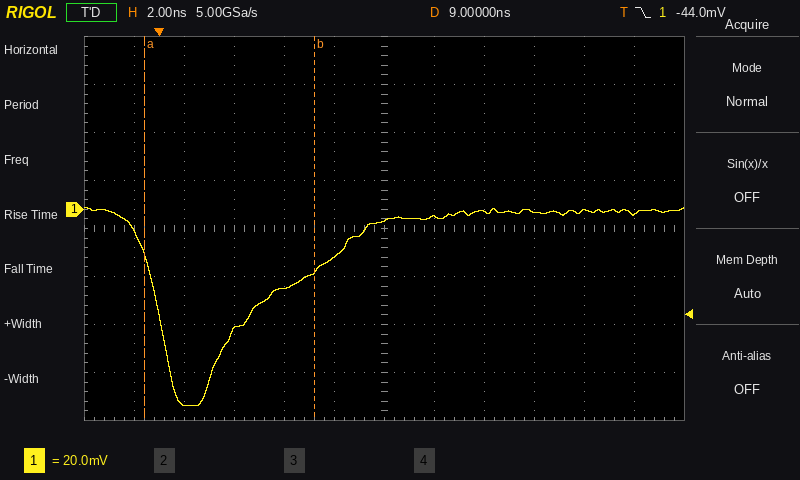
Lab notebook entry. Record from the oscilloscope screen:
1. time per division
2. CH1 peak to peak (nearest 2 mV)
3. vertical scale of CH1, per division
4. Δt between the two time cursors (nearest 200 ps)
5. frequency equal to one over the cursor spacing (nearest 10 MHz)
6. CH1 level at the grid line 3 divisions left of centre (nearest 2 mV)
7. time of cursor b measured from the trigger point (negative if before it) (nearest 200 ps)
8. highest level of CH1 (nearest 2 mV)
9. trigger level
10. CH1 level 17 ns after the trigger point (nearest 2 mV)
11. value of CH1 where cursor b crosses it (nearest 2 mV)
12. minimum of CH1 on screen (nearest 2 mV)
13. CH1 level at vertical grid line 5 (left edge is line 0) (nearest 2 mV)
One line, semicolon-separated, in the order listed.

2 ns; 82 mV; 20 mV; 6.8 ns; 150 MHz; -50 mV; +6.2 ns; 0 mV; -44.0 mV; 0 mV; -26 mV; -82 mV; -20 mV
